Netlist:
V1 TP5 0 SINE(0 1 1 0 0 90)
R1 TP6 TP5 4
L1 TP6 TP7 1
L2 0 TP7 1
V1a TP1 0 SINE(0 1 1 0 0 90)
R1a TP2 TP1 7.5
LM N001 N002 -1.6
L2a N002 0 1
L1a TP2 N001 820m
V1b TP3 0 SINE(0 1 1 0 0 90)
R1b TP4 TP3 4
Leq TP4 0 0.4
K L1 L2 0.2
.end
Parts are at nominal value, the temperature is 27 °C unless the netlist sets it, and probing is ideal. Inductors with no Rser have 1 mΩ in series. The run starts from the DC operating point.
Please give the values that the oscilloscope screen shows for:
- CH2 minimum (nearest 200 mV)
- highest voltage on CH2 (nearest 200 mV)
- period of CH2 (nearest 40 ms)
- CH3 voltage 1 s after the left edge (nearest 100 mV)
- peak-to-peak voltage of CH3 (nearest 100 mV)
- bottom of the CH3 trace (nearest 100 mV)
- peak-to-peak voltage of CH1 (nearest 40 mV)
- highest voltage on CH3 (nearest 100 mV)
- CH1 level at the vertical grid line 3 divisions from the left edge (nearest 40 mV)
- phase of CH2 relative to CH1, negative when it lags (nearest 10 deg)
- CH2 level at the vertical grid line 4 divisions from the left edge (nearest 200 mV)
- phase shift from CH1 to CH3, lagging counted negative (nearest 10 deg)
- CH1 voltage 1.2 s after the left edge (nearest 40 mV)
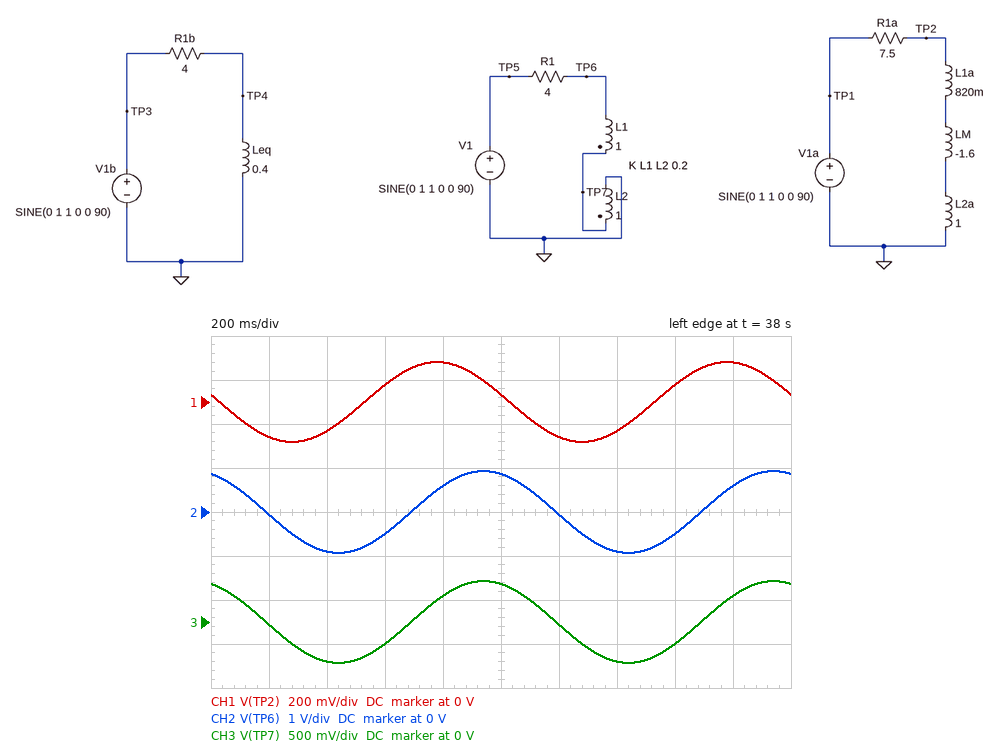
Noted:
-1.0 V
1.0 V
1.00 s
400 mV
900 mV
-500 mV
360 mV
500 mV
80 mV
-60 deg
600 mV
-60 deg
-160 mV
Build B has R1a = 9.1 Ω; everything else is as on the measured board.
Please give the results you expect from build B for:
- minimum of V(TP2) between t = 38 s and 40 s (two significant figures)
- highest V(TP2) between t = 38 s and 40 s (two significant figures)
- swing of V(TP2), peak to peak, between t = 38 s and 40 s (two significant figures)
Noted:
-150 mV
150 mV
300 mV
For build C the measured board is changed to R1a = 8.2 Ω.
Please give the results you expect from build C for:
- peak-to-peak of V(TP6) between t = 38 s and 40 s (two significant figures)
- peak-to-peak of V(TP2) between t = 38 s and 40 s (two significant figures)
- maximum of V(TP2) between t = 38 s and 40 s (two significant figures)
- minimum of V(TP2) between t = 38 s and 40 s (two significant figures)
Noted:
1.9 V
330 mV
170 mV
-170 mV
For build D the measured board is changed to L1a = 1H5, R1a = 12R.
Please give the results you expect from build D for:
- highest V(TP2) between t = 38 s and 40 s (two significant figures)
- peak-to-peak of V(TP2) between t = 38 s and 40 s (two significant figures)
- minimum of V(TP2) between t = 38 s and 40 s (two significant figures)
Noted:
430 mV
850 mV
-430 mV
